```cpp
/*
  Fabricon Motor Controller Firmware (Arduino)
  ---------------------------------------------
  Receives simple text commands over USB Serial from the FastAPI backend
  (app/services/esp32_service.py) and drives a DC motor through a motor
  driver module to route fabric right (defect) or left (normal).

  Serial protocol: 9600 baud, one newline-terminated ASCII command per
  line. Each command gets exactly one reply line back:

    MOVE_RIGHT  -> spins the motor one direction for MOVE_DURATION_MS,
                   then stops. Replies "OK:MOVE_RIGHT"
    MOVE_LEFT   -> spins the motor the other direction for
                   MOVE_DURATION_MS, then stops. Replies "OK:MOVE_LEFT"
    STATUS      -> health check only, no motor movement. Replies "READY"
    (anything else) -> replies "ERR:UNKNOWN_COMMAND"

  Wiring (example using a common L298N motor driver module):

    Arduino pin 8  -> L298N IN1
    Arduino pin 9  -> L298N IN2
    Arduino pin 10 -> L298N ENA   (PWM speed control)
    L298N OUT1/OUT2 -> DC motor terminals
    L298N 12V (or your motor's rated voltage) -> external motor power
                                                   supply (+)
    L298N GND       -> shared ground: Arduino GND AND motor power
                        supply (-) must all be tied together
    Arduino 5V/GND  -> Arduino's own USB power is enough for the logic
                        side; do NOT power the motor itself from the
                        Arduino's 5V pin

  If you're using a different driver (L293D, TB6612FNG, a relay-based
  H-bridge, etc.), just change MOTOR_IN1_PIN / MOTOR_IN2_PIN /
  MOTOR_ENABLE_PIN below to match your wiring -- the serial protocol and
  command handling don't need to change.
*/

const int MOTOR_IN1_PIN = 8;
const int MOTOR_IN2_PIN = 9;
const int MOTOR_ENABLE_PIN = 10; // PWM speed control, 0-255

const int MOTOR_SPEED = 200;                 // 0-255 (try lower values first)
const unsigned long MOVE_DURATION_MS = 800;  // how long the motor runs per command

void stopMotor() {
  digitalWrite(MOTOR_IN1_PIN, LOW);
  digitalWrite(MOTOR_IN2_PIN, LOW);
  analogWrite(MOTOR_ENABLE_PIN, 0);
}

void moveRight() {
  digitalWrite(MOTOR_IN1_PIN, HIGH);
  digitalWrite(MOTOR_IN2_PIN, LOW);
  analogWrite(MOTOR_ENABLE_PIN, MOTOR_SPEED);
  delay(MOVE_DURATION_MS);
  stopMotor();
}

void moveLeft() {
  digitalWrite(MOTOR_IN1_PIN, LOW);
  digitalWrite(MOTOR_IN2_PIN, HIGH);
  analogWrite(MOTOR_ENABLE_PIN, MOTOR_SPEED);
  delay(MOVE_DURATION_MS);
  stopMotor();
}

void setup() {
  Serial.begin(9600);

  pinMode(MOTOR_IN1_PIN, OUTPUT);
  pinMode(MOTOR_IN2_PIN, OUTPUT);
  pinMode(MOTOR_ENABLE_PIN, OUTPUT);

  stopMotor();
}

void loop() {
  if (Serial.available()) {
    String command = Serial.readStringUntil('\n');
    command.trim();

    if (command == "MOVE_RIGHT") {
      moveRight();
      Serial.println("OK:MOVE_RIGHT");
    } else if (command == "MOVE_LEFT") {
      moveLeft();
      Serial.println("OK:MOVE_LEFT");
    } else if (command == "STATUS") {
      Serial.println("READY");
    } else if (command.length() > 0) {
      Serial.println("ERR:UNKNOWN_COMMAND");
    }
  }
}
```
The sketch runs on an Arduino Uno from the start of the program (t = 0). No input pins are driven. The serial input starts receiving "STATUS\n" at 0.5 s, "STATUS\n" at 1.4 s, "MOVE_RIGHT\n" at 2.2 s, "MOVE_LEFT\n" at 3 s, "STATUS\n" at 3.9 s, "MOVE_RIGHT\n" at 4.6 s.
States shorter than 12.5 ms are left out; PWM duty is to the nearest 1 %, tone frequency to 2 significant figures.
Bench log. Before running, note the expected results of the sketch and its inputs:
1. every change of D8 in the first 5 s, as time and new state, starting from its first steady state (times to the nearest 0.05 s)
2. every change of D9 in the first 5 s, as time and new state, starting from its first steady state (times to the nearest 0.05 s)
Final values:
0 s low; 2.2 s high; 3 s low; 4.6 s high
0 s low; 3 s high; 3.8 s low
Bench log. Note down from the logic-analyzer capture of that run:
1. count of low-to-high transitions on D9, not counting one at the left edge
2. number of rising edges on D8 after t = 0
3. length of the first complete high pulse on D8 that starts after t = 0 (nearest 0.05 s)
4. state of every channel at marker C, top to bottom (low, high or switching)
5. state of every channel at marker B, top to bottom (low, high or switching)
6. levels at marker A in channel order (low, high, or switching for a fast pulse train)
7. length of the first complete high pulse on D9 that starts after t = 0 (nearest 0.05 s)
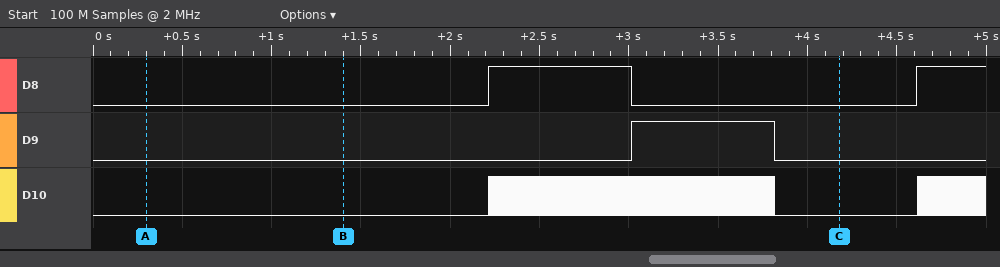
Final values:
1
2
0.80 s
D8 low, D9 low, D10 low
D8 low, D9 low, D10 low
D8 low, D9 low, D10 low
0.80 s
